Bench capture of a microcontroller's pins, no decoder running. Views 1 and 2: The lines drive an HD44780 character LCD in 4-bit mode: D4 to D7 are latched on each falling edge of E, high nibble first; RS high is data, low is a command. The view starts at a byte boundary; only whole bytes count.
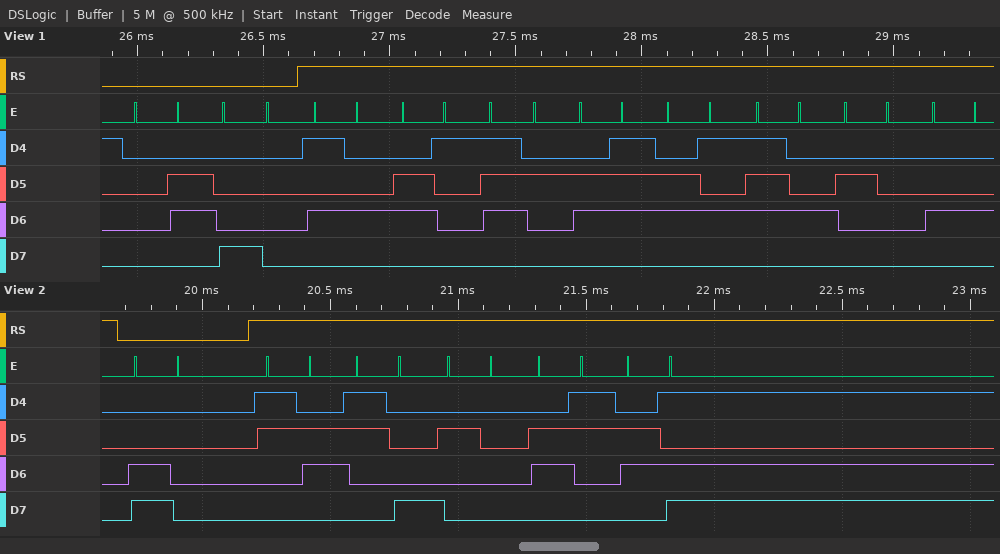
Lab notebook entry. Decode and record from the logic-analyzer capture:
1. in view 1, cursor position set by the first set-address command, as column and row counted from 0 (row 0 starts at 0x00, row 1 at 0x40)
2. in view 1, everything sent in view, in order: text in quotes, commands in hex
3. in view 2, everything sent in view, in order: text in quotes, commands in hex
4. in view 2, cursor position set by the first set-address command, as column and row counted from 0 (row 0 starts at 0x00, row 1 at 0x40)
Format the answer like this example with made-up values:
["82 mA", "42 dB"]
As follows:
["column 0, row 0", "0x06 0x80 \"Target D\"", "0xC0 \"68 cm\"", "column 0, row 1"]
